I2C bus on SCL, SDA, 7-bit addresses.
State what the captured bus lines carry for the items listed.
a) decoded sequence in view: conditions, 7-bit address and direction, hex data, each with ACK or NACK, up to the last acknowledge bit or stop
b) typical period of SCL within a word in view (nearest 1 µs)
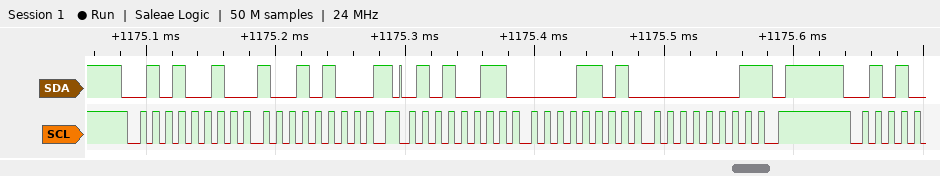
start, address 29 write ACK, 94 ACK, repeated start, address 29 read ACK, 0D ACK, 01 NACK, stop
10 µs
